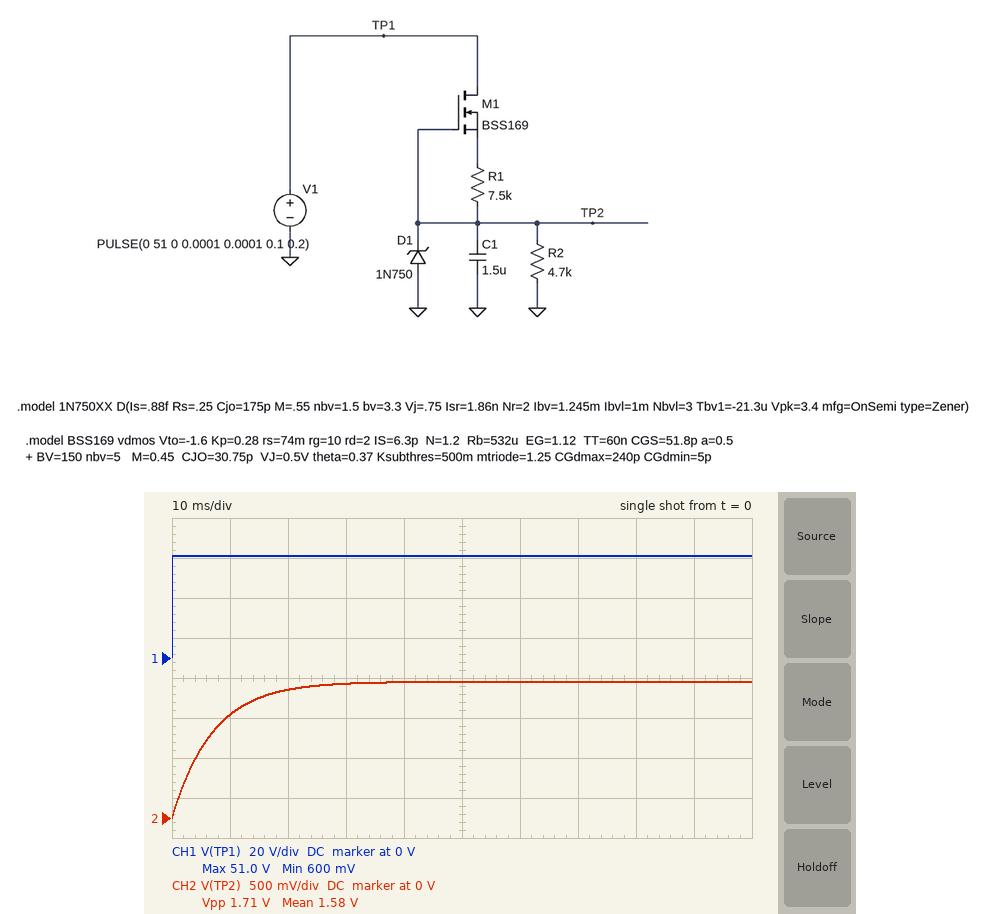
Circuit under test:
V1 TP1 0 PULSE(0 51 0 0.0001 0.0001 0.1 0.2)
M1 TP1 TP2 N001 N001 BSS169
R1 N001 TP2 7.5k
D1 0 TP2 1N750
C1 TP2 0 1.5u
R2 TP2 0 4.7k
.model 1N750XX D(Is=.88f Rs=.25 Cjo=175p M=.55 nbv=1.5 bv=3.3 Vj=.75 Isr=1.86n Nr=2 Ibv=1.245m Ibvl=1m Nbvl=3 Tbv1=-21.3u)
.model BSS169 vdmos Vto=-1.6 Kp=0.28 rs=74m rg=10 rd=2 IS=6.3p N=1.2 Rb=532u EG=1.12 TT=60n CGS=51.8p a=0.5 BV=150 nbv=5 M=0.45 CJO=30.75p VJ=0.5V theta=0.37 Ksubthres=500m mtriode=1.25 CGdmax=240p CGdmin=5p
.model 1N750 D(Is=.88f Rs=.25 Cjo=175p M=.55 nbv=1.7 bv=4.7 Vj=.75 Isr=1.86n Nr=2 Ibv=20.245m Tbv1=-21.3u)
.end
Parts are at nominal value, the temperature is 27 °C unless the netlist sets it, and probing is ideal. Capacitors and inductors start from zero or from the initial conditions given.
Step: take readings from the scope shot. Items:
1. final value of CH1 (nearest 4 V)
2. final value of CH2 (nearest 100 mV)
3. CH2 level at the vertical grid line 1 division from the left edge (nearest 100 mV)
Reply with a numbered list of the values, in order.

1. 52 V
2. 1.7 V
3. 1.3 V
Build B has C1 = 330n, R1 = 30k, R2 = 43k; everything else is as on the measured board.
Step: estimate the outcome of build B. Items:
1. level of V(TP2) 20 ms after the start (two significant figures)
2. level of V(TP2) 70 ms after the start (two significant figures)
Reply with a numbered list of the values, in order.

1. 3.3 V
2. 4.3 V
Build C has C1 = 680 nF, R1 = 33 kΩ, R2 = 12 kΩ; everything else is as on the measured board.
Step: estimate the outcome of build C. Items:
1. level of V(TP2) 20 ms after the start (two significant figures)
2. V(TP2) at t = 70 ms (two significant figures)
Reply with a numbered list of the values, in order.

1. 1.0 V
2. 1.1 V
